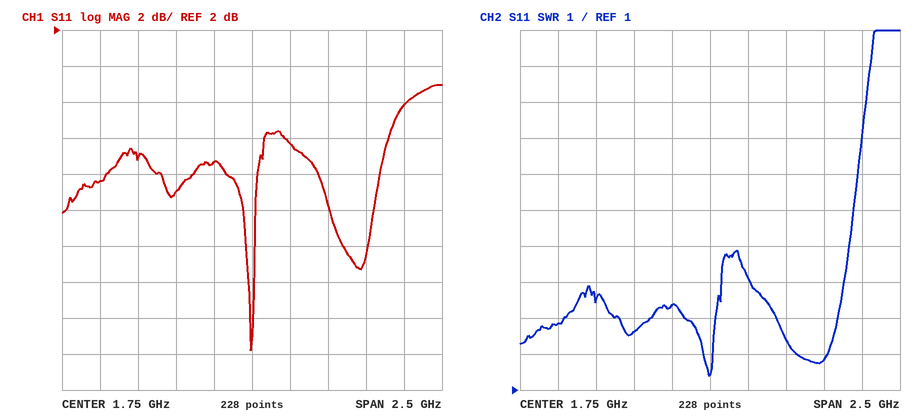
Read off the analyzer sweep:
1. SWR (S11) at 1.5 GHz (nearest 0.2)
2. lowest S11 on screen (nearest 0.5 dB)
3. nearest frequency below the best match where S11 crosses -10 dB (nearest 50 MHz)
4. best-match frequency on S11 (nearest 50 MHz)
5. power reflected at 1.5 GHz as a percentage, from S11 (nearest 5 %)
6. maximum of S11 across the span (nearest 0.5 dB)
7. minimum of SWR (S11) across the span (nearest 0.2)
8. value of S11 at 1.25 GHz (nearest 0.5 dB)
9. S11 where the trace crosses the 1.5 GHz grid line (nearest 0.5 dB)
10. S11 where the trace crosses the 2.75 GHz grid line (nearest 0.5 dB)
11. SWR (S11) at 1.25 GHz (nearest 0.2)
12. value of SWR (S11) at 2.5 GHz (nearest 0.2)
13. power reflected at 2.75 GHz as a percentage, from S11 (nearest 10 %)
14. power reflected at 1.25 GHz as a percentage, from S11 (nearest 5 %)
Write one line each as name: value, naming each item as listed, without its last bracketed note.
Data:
SWR (S11) at 1.5 GHz: 3.4
lowest S11 on screen: -16.0 dB
nearest frequency below the best match where S11 crosses -10 dB: 1.70 GHz
best-match frequency on S11: 1.75 GHz
power reflected at 1.5 GHz as a percentage, from S11: 30 %
maximum of S11 across the span: -1.0 dB
minimum of SWR (S11) across the span: 1.4
value of S11 at 1.25 GHz: -7.0 dB
S11 where the trace crosses the 1.5 GHz grid line: -5.5 dB
S11 where the trace crosses the 2.75 GHz grid line: -2.0 dB
SWR (S11) at 1.25 GHz: 2.6
value of SWR (S11) at 2.5 GHz: 1.8
power reflected at 2.75 GHz as a percentage, from S11: 60 %
power reflected at 1.25 GHz as a percentage, from S11: 20 %
